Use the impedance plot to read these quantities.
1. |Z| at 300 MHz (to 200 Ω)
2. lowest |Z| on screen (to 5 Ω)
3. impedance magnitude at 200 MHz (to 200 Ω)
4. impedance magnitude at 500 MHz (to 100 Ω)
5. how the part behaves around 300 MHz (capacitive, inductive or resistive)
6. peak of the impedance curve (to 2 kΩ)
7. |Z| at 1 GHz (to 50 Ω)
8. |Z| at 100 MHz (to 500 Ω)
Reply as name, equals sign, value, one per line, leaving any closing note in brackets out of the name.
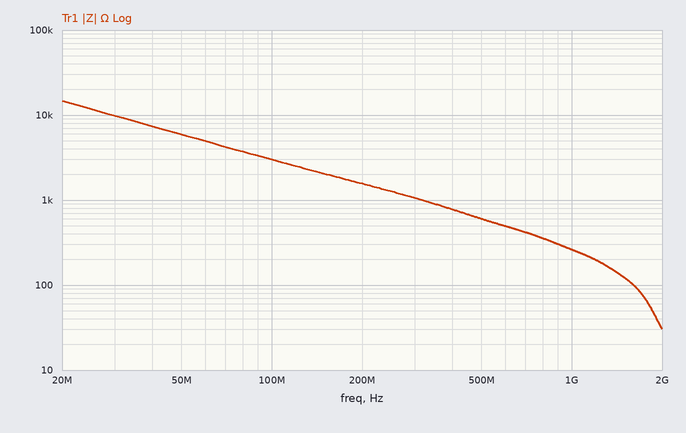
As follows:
|Z| at 300 MHz = 1.0 kΩ
lowest |Z| on screen = 30 Ω
impedance magnitude at 200 MHz = 1.6 kΩ
impedance magnitude at 500 MHz = 600 Ω
how the part behaves around 300 MHz = capacitive
peak of the impedance curve = 14 kΩ
|Z| at 1 GHz = 250 Ω
|Z| at 100 MHz = 3.0 kΩ
